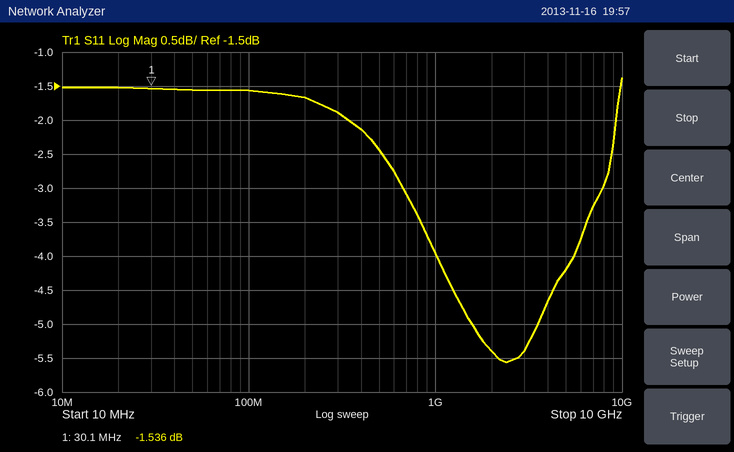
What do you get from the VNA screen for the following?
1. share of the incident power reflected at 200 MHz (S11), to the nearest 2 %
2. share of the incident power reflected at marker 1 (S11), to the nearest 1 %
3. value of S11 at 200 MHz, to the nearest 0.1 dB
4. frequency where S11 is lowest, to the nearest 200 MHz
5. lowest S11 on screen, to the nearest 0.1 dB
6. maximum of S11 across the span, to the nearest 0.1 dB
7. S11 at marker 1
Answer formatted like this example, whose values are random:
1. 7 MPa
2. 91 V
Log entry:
1. 68 %
2. 70 %
3. -1.7 dB
4. 2.4 GHz
5. -5.6 dB
6. -1.4 dB
7. -1.536 dB
